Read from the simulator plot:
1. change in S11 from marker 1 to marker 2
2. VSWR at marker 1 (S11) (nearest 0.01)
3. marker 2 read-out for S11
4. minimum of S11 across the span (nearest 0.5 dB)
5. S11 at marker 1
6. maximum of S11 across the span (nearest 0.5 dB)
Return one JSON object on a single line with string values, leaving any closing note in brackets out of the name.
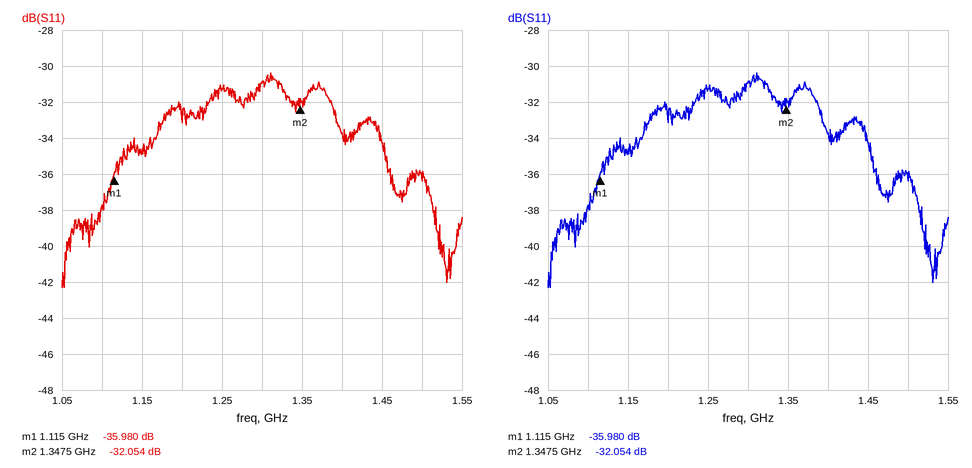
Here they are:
{"change in S11 from marker 1 to marker 2": "3.926 dB", "VSWR at marker 1 (S11)": "1.03", "marker 2 read-out for S11": "-32.054 dB", "minimum of S11 across the span": "-42.5 dB", "S11 at marker 1": "-35.980 dB", "maximum of S11 across the span": "-30.5 dB"}
